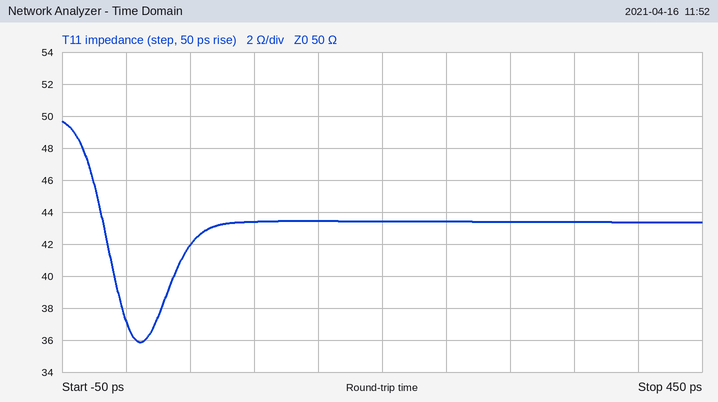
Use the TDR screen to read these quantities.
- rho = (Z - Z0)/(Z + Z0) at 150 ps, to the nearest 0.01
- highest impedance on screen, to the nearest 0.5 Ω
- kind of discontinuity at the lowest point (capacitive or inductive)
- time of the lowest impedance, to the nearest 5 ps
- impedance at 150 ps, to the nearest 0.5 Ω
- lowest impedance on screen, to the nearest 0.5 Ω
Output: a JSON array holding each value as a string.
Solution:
["-0.07", "49.5 Ω", "capacitive", "10 ps", "43.5 Ω", "36.0 Ω"]
